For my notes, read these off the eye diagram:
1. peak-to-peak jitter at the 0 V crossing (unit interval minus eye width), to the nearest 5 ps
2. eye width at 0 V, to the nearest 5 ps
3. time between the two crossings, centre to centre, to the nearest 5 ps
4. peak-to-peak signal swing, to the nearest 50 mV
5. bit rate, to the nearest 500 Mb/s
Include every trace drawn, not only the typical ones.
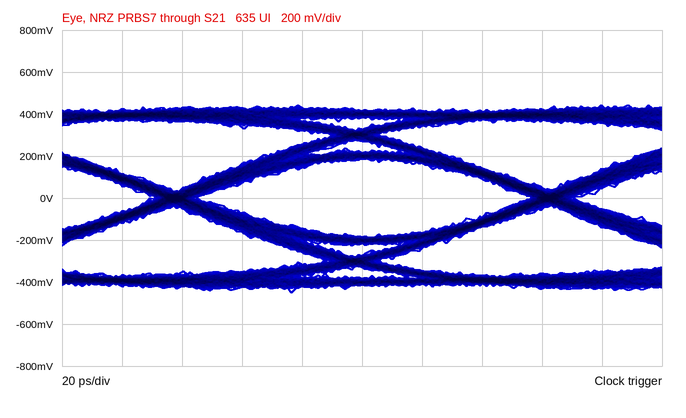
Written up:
15 ps
110 ps
125 ps
900 mV
8.0 Gb/s
